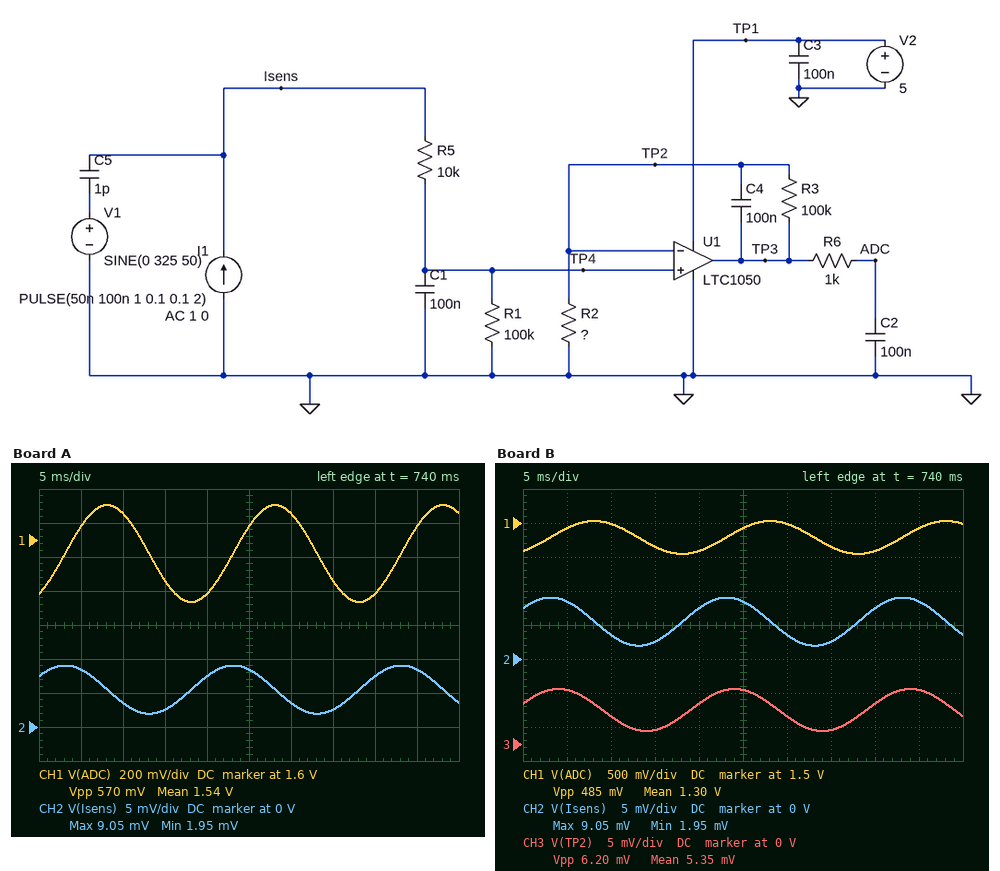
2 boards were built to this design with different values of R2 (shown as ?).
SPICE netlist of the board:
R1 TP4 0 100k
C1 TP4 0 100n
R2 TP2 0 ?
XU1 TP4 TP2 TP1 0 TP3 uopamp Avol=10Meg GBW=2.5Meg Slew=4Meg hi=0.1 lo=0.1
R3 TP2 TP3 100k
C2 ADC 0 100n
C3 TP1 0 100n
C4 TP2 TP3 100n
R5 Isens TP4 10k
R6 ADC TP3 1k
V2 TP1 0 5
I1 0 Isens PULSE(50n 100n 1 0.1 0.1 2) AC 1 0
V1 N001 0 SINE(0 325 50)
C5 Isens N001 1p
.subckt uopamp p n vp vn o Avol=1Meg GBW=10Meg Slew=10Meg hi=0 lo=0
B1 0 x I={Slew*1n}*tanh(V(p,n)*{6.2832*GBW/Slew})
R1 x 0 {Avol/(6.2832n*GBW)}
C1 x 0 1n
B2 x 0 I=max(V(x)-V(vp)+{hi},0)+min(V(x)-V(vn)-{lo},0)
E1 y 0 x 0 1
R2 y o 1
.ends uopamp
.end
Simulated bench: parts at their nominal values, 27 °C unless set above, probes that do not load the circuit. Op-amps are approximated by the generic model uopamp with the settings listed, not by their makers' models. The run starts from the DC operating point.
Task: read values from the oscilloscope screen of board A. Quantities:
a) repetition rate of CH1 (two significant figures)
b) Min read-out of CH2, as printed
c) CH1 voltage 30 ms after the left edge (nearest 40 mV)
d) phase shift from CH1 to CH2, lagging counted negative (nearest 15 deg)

50 Hz
1.95 mV
1.76 V
90 deg
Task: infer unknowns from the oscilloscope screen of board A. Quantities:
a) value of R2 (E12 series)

330 Ω
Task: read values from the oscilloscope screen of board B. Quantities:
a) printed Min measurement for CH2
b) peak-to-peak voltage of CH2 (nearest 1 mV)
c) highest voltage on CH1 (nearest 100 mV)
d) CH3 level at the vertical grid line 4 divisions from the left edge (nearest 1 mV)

1.95 mV
7 mV
1.5 V
6 mV
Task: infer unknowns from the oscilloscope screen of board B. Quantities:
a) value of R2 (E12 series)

390 Ω
